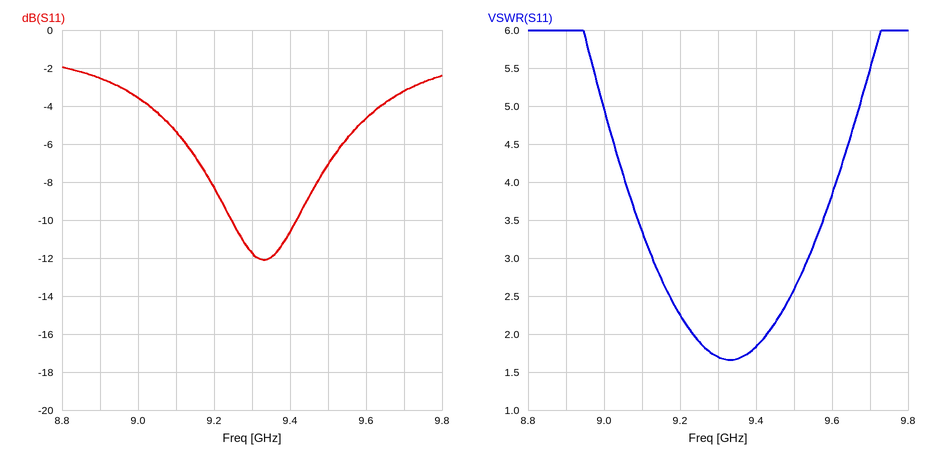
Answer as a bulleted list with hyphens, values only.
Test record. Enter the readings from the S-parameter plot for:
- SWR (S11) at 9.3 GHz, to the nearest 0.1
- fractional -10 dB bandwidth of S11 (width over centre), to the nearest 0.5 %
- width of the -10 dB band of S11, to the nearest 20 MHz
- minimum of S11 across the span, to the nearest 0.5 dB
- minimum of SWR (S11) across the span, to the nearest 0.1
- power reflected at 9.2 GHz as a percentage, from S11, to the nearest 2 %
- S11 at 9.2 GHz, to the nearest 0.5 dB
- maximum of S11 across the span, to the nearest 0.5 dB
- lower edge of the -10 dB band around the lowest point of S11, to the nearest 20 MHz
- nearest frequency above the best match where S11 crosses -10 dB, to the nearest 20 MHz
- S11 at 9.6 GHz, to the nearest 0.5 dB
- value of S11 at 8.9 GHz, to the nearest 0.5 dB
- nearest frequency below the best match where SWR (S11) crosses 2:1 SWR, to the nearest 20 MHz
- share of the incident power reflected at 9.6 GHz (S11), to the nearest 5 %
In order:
- 1.7
- 2.0 %
- 180 MHz
- -12.0 dB
- 1.7
- 14 %
- -8.5 dB
- -2.0 dB
- 9.24 GHz
- 9.42 GHz
- -4.5 dB
- -2.5 dB
- 9.24 GHz
- 35 %
